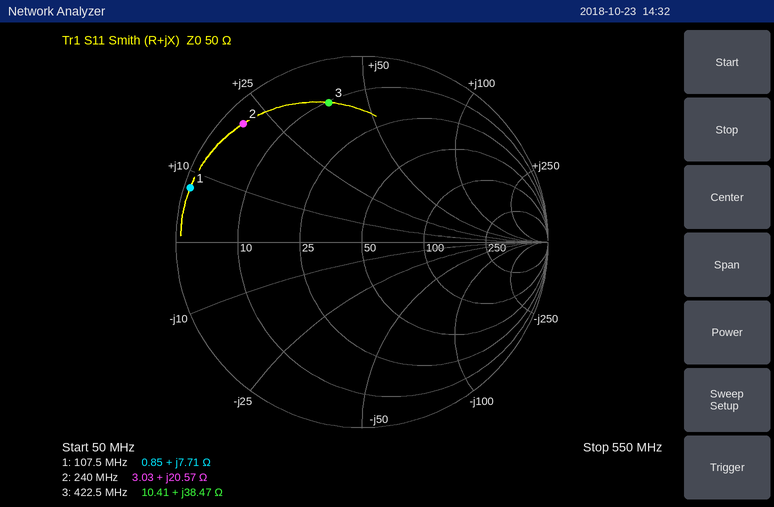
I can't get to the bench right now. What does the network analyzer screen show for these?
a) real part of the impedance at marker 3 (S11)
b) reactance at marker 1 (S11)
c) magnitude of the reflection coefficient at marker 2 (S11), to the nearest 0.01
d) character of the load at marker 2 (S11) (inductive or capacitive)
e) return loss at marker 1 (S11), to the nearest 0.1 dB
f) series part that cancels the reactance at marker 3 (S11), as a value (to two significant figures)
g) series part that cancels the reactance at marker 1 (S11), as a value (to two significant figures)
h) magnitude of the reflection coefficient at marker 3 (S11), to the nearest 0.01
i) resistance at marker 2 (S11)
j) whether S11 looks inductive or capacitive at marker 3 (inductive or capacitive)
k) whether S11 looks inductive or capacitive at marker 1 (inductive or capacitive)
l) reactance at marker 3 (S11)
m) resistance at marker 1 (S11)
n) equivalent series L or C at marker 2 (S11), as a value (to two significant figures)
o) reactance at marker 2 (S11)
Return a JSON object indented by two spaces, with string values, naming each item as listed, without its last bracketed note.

{
  "real part of the impedance at marker 3": "10.41 Ω",
  "reactance at marker 1": "+7.71 Ω",
  "magnitude of the reflection coefficient at marker 2 (S11), to the nearest 0.01": "0.90",
  "character of the load at marker 2 (S11)": "inductive",
  "return loss at marker 1 (S11), to the nearest 0.1 dB": "0.3 dB",
  "series part that cancels the reactance at marker 3 (S11), as a value": "9.8 pF",
  "series part that cancels the reactance at marker 1 (S11), as a value": "190 pF",
  "magnitude of the reflection coefficient at marker 3 (S11), to the nearest 0.01": "0.77",
  "resistance at marker 2": "3.03 Ω",
  "whether S11 looks inductive or capacitive at marker 3": "inductive",
  "whether S11 looks inductive or capacitive at marker 1": "inductive",
  "reactance at marker 3": "+38.47 Ω",
  "resistance at marker 1": "0.85 Ω",
  "equivalent series L or C at marker 2 (S11), as a value": "14 nH",
  "reactance at marker 2": "+20.57 Ω"
}
